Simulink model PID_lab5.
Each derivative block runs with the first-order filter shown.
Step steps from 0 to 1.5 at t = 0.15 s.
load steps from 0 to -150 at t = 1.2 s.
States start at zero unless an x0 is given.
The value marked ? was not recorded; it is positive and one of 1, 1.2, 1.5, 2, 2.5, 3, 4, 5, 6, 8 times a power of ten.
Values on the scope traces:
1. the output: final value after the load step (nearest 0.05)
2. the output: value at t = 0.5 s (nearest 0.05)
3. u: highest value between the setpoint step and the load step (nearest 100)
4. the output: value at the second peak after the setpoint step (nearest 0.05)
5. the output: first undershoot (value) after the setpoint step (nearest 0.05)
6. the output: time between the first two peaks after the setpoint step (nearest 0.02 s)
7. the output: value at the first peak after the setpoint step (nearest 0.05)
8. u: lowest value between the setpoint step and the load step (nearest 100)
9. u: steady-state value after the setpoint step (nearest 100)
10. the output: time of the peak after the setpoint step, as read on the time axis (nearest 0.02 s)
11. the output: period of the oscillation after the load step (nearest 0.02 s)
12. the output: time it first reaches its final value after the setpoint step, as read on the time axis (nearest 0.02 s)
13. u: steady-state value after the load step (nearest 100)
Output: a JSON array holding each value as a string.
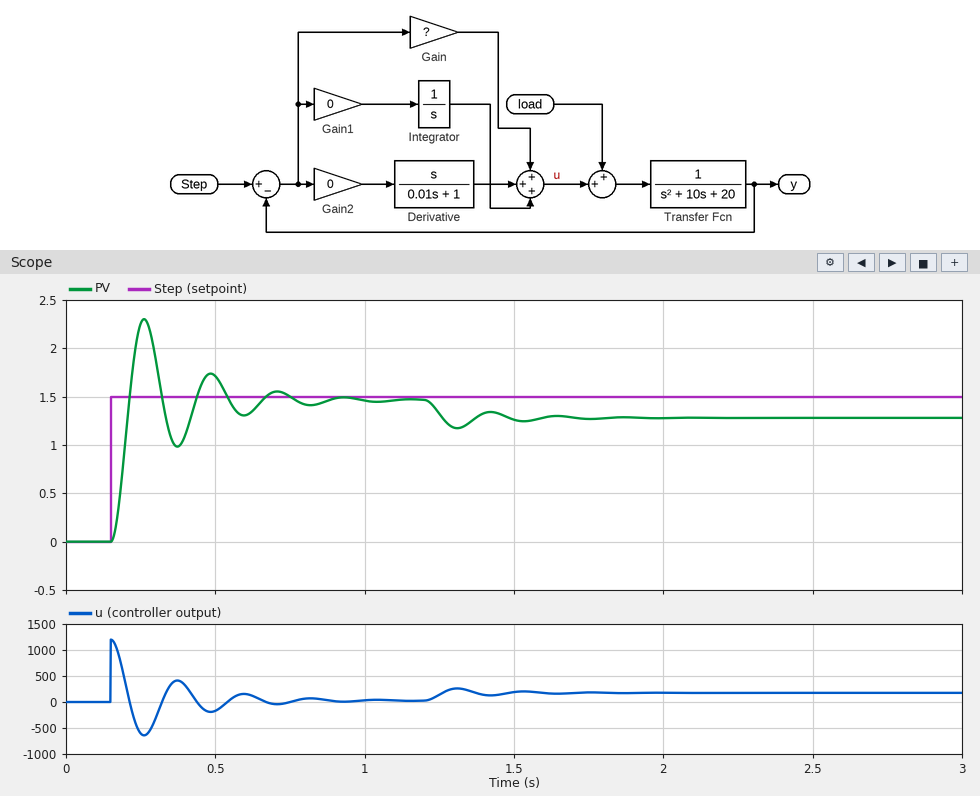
["1.30", "1.70", "1200", "1.75", "1.00", "0.22 s", "2.30", "-600", "0", "0.26 s", "0.22 s", "0.22 s", "200"]
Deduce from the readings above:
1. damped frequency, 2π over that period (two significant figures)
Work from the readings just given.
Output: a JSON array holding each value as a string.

["29 rad/s"]
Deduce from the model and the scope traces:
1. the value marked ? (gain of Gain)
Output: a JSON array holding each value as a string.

["800"]
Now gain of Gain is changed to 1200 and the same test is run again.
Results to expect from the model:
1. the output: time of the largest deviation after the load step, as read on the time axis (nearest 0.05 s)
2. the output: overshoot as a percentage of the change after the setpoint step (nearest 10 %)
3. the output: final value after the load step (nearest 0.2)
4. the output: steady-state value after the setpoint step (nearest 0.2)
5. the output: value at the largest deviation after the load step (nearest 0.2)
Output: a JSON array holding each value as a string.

["1.30 s", "60 %", "1.4", "1.4", "1.2"]
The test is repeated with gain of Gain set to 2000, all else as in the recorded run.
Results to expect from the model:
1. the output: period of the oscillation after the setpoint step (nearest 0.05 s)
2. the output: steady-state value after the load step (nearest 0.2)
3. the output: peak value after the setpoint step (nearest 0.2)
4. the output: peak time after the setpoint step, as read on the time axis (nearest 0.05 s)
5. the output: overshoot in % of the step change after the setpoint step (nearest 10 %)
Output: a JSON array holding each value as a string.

["0.15 s", "1.4", "2.6", "0.20 s", "70 %"]
